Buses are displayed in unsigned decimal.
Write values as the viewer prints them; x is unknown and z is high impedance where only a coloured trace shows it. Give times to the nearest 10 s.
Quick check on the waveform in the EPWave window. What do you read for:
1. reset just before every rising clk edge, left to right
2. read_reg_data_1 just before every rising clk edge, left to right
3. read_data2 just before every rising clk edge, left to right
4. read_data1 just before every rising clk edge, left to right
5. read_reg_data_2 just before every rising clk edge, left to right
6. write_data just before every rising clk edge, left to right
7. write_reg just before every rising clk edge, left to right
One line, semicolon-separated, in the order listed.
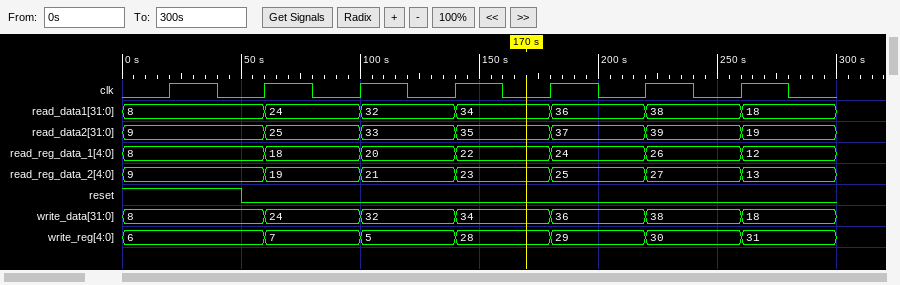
1 0 0 0 0 0 0; 8, 8, 18, 20, 22, 24, 26; 9, 9, 25, 33, 35, 37, 39; 8, 8, 24, 32, 34, 36, 38; 9, 9, 19, 21, 23, 25, 27; 8, 8, 24, 32, 34, 36, 38; 6, 6, 7, 5, 28, 29, 30
